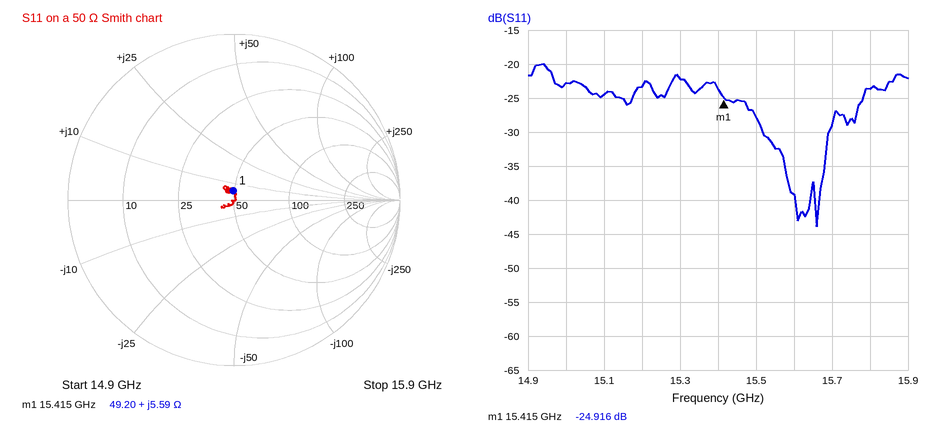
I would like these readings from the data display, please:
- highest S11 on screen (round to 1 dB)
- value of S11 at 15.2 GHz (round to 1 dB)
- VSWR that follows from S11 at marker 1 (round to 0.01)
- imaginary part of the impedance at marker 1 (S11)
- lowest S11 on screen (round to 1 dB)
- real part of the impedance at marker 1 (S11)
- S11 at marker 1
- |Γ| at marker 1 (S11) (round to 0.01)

-20 dB
-23 dB
1.12
+5.59 Ω
-44 dB
49.20 Ω
-24.916 dB
0.06
